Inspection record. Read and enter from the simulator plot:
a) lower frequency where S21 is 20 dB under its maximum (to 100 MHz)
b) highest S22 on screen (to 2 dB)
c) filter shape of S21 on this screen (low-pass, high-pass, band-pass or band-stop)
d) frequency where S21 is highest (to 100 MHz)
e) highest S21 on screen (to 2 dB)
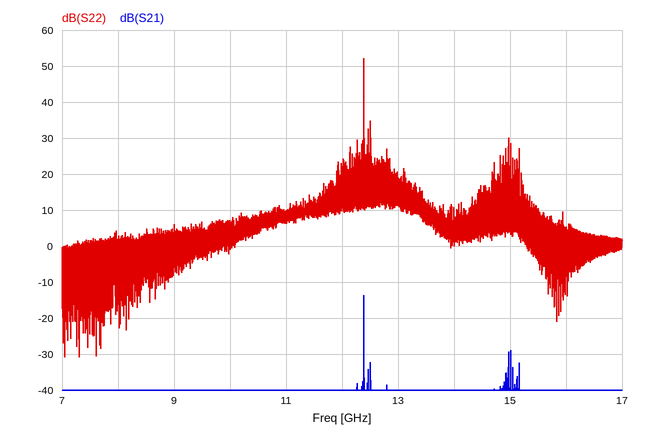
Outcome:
12.4 GHz
52 dB
band-pass
12.4 GHz
-14 dB
